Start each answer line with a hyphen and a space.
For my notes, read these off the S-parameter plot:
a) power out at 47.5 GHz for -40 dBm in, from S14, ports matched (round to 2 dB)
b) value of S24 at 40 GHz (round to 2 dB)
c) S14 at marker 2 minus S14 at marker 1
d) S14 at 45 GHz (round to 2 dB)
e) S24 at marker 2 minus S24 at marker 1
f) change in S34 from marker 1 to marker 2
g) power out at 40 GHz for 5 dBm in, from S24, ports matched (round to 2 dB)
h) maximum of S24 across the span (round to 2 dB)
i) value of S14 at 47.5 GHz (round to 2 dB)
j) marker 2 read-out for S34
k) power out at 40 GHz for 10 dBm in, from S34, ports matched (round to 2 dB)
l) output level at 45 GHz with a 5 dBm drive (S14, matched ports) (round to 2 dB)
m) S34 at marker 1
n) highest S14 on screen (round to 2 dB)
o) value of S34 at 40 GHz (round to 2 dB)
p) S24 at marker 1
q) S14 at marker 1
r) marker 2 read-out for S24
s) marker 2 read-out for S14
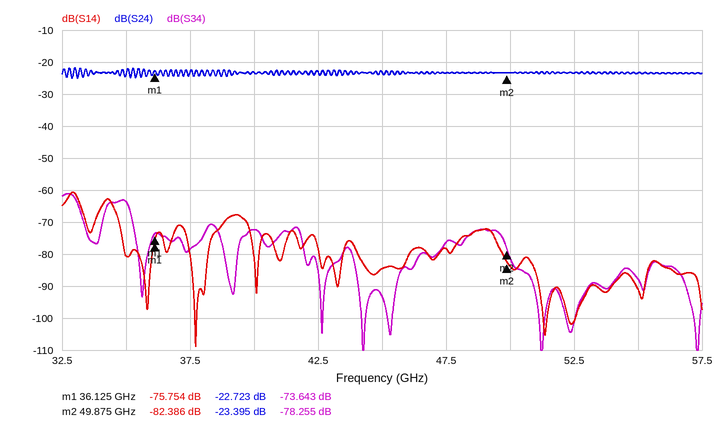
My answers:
- -118 dBm
- -24 dB
- -6.632 dB
- -84 dB
- -0.672 dB
- -4.612 dB
- -18 dBm
- -22 dB
- -78 dB
- -78.255 dB
- -62 dBm
- -80 dBm
- -73.643 dB
- -60 dB
- -72 dB
- -22.723 dB
- -75.754 dB
- -23.395 dB
- -82.386 dB
